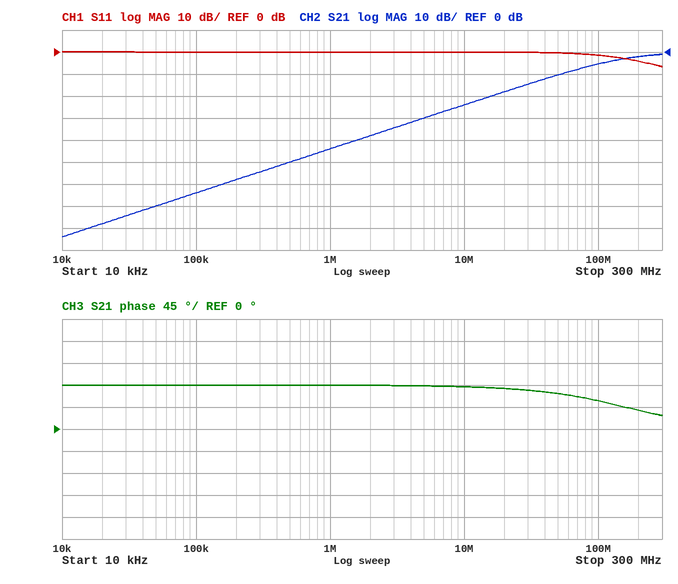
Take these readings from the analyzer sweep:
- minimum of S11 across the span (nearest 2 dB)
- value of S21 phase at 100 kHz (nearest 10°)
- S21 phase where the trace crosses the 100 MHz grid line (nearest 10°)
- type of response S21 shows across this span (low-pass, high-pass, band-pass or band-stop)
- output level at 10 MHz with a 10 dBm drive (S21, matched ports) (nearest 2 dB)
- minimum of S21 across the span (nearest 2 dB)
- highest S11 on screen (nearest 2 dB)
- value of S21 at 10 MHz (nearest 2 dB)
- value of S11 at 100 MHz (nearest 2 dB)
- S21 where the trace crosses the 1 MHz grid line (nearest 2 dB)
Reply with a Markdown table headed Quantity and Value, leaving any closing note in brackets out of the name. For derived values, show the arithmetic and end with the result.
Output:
| Quantity | Value |
|---|---|
| minimum of S11 across the span | -6 dB |
| value of S21 phase at 100 kHz | 90° |
| S21 phase where the trace crosses the 100 MHz grid line | 60° |
| type of response S21 shows across this span | high-pass |
| output level at 10 MHz with a 10 dBm drive (S21, matched ports) | 10 dBm + (-24 dB) = -14 dBm |
| minimum of S21 across the span | -84 dB |
| highest S11 on screen | 0 dB |
| value of S21 at 10 MHz | -24 dB |
| value of S11 at 100 MHz | -2 dB |
| S21 where the trace crosses the 1 MHz grid line | -44 dB |
